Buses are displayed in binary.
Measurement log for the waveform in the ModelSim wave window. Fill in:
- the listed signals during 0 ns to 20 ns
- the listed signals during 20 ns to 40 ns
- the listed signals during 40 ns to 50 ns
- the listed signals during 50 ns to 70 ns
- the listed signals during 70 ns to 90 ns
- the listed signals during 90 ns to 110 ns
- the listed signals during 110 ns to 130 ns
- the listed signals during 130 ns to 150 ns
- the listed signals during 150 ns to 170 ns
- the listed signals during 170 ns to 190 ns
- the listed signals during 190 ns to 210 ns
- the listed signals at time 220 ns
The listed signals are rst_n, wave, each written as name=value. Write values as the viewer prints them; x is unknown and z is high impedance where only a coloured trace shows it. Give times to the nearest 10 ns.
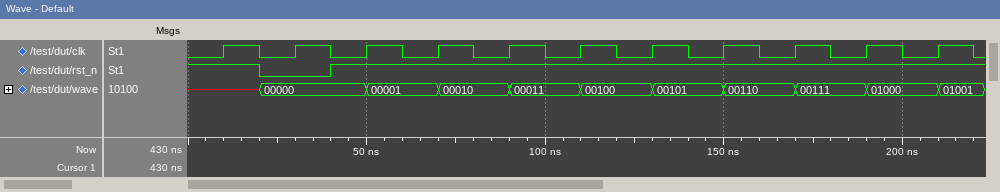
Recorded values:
rst_n=1, wave=x
rst_n=0, wave=00000
rst_n=1, wave=00000
rst_n=1, wave=00001
rst_n=1, wave=00010
rst_n=1, wave=00011
rst_n=1, wave=00100
rst_n=1, wave=00101
rst_n=1, wave=00110
rst_n=1, wave=00111
rst_n=1, wave=01000
rst_n=1, wave=01001
